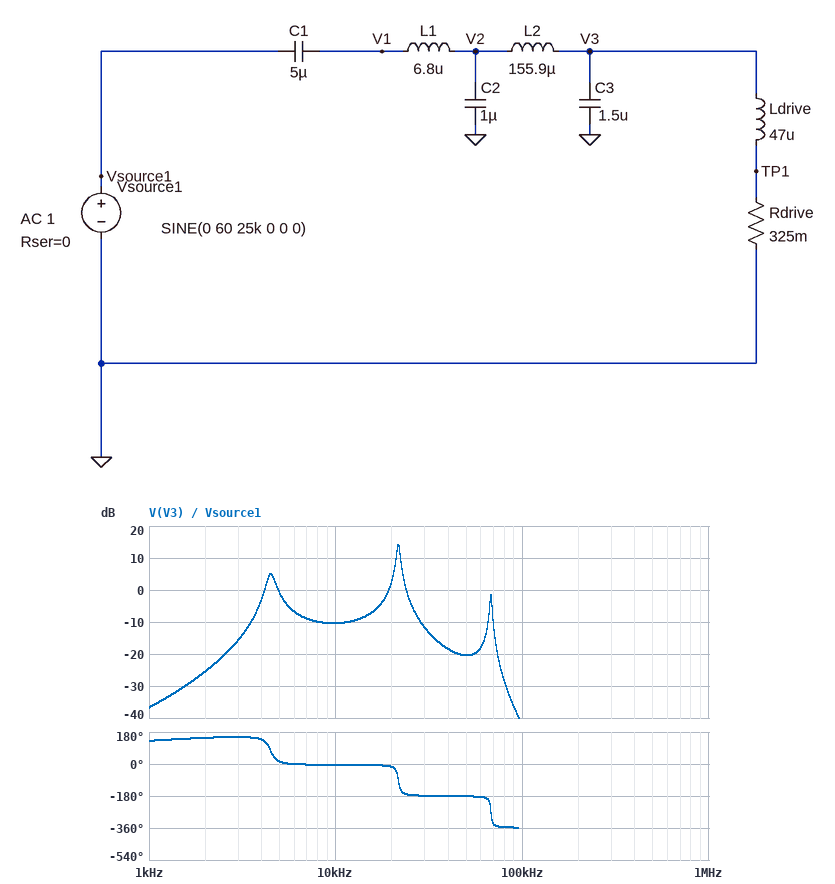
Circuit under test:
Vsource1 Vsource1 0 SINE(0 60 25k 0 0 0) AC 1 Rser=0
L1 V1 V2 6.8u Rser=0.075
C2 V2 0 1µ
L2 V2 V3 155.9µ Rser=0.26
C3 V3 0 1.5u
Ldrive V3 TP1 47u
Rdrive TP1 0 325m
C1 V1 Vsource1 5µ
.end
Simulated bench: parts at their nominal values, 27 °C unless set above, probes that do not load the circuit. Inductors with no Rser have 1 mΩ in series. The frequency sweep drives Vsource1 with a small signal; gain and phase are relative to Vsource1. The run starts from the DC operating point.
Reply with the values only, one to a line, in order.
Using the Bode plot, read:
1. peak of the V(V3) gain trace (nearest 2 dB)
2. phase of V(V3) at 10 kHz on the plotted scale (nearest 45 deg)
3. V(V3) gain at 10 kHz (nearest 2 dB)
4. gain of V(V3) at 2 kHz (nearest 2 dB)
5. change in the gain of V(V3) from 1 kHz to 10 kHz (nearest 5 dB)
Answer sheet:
14 dB
0 deg
-10 dB
-26 dB
25 dB
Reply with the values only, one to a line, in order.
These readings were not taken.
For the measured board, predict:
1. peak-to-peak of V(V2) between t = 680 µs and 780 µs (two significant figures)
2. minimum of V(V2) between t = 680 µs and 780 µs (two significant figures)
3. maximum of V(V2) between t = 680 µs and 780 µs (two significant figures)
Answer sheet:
120 V
-62 V
58 V
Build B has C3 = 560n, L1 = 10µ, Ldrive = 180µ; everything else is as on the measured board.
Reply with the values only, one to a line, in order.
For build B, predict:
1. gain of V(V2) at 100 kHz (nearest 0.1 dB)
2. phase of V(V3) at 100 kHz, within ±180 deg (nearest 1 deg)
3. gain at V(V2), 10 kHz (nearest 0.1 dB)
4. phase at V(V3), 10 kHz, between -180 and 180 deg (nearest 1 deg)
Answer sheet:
-8.6 dB
1 deg
-0.6 dB
0 deg
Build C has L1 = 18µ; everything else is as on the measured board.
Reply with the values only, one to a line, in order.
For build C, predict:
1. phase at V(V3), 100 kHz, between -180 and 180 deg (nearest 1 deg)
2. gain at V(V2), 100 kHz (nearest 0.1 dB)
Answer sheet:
1 deg
-15.3 dB
